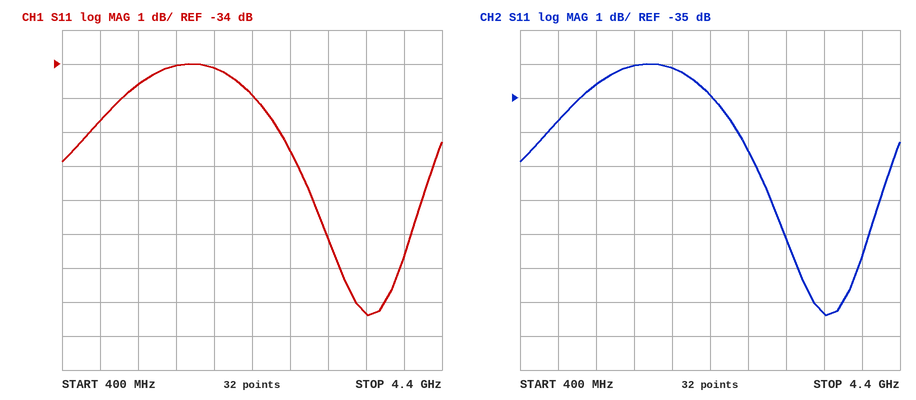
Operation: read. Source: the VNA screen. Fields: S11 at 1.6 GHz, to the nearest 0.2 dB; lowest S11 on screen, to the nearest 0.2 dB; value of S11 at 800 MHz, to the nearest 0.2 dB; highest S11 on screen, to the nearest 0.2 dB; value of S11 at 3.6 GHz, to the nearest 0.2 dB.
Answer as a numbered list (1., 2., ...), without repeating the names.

1. -34.0 dB
2. -41.4 dB
3. -35.6 dB
4. -34.0 dB
5. -41.4 dB
